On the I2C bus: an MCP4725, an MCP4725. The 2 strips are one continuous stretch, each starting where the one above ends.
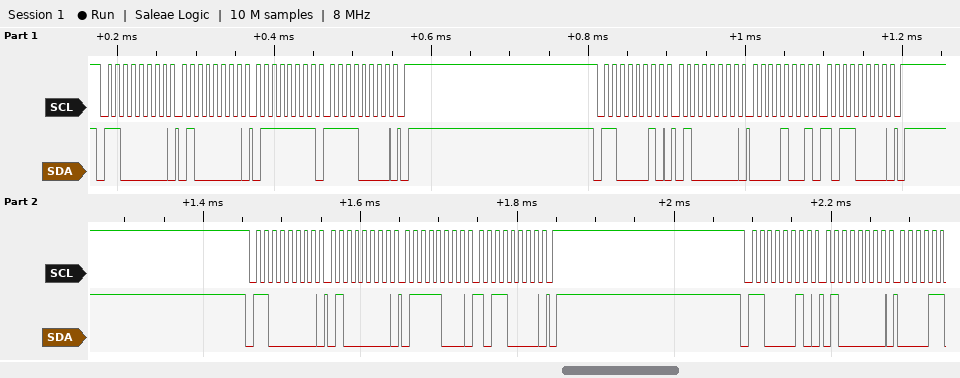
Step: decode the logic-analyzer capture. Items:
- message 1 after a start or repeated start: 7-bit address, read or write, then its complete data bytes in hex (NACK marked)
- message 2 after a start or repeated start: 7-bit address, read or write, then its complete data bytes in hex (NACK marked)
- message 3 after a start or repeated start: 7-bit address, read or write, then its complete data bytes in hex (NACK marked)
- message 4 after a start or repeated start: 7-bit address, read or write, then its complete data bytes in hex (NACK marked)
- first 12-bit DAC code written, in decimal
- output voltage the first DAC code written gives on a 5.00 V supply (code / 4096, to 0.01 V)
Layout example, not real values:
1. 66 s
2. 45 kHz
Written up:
1. 0x60 write: 40 7F F0
2. 0x61 write: 40 09 B0
3. 0x60 write: 40 78 B0
4. 0x61 write: 40
5. 2047
6. 2.50 V
